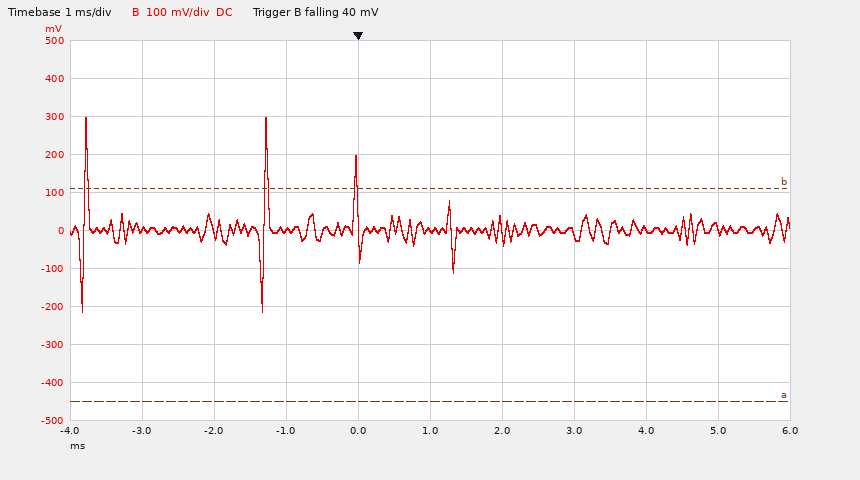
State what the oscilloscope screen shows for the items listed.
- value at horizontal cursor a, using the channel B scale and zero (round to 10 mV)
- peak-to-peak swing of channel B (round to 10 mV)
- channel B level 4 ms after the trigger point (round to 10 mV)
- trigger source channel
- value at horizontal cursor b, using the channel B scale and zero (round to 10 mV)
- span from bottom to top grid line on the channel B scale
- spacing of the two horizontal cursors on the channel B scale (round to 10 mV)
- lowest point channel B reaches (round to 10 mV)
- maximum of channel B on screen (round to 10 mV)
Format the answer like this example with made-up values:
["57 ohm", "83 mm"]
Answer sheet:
["-450 mV", "510 mV", "0 mV", "channel B", "110 mV", "1 V", "560 mV", "-210 mV", "300 mV"]
